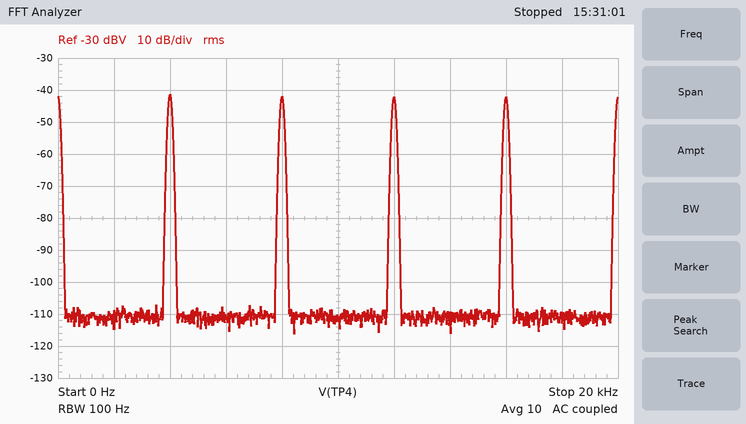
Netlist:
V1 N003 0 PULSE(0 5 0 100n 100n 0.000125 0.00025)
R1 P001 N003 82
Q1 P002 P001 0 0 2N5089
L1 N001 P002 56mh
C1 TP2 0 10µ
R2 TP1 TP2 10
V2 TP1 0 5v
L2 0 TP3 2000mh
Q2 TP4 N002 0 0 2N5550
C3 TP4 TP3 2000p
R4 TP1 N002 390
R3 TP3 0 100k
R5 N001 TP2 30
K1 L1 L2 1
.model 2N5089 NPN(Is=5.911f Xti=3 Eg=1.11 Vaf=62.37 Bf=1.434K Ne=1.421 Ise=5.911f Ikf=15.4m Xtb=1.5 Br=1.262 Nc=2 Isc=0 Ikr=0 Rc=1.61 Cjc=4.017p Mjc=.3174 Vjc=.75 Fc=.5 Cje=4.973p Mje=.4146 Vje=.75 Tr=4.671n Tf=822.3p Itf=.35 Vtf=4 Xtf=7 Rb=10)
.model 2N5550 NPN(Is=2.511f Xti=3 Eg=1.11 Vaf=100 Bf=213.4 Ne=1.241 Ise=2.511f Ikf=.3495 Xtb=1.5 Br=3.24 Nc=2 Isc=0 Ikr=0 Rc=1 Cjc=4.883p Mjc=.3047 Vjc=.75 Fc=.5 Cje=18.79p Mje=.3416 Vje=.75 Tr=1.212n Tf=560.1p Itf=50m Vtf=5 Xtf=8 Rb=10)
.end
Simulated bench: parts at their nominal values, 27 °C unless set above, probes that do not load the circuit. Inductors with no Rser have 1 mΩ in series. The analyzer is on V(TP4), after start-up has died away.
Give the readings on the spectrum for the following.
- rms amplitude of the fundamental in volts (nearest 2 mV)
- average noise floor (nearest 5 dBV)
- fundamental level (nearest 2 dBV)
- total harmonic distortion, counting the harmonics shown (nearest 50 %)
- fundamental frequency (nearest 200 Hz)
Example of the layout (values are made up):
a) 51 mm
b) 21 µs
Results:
a) 8 mV
b) -110 dBV
c) -42 dBV
d) 150 %
e) 4.0 kHz
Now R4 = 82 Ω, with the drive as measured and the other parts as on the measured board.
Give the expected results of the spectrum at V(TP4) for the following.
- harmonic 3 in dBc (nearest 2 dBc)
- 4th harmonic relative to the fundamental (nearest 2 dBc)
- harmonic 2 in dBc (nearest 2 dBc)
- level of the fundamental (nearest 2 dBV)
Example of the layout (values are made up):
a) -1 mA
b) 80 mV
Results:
a) -4 dBc
b) -4 dBc
c) -4 dBc
d) -56 dBV
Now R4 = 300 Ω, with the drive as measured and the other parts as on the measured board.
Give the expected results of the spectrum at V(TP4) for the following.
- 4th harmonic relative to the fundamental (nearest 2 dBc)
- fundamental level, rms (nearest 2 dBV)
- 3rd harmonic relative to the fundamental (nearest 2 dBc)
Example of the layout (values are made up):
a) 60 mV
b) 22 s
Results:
a) -2 dBc
b) -50 dBV
c) -2 dBc
